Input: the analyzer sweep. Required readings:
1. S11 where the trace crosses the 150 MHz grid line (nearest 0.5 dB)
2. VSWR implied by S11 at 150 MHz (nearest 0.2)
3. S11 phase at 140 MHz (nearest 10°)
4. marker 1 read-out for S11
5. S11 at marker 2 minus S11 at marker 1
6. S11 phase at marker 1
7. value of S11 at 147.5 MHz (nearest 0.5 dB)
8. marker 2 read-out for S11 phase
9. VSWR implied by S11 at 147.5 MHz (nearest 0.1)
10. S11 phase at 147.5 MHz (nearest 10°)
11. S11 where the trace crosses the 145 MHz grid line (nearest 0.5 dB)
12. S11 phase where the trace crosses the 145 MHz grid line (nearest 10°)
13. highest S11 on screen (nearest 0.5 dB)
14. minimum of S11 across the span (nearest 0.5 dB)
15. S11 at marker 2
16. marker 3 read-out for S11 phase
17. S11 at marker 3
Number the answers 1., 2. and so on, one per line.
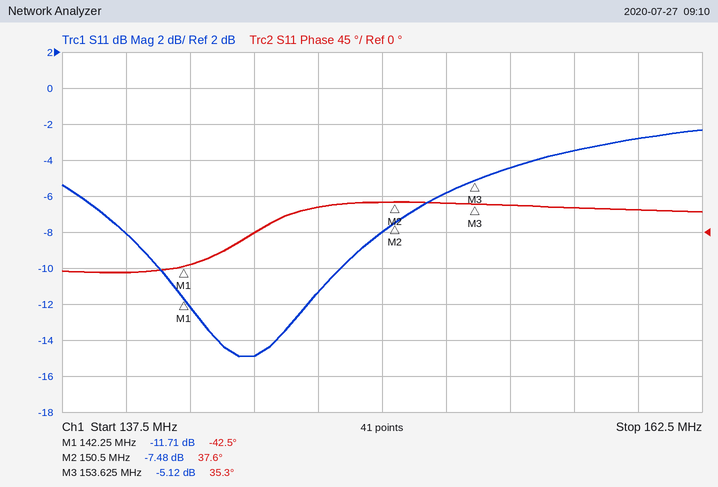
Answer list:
1. -8.0 dB
2. 2.4
3. -50°
4. -11.71 dB
5. 4.23 dB
6. -42.5°
7. -11.5 dB
8. 37.6°
9. 1.7
10. 30°
11. -15.0 dB
12. 0°
13. -2.5 dB
14. -15.0 dB
15. -7.48 dB
16. 35.3°
17. -5.12 dB
